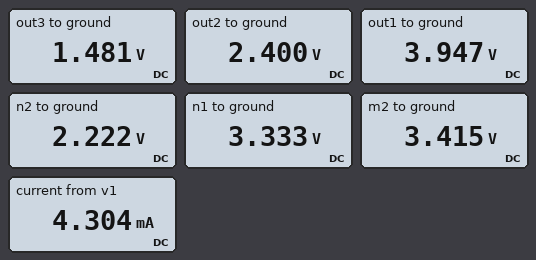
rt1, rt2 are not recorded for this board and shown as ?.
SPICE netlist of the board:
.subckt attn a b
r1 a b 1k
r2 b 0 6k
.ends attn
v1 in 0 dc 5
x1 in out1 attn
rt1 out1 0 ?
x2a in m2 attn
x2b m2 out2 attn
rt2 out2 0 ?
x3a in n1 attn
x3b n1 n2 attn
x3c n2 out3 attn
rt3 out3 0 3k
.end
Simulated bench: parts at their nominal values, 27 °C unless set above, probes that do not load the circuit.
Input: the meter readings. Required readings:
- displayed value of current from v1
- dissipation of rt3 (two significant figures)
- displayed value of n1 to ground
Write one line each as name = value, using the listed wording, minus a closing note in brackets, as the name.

displayed value of current from v1 = 4.304 mA
dissipation of rt3 = 730 µW
displayed value of n1 to ground = 3.333 V
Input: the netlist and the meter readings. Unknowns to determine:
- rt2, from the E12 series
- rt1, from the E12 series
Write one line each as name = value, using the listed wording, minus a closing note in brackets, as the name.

rt2, from the E12 series = 3.9 kΩ
rt1, from the E12 series = 10 kΩ
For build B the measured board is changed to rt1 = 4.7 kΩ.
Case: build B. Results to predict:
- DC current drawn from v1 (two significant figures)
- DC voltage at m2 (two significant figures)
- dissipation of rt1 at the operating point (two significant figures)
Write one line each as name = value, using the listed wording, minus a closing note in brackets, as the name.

DC current drawn from v1 = 4.6 mA
DC voltage at m2 = 3.4 V
dissipation of rt1 at the operating point = 2.8 mW
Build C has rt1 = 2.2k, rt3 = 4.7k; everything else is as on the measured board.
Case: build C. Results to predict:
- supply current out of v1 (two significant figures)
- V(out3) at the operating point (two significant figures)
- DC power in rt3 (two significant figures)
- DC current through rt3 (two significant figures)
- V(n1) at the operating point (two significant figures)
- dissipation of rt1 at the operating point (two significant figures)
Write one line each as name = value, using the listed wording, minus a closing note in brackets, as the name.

supply current out of v1 = 5.1 mA
V(out3) at the operating point = 1.7 V
DC power in rt3 = 620 µW
DC current through rt3 = 360 µA
V(n1) at the operating point = 3.4 V
dissipation of rt1 at the operating point = 4.3 mW
